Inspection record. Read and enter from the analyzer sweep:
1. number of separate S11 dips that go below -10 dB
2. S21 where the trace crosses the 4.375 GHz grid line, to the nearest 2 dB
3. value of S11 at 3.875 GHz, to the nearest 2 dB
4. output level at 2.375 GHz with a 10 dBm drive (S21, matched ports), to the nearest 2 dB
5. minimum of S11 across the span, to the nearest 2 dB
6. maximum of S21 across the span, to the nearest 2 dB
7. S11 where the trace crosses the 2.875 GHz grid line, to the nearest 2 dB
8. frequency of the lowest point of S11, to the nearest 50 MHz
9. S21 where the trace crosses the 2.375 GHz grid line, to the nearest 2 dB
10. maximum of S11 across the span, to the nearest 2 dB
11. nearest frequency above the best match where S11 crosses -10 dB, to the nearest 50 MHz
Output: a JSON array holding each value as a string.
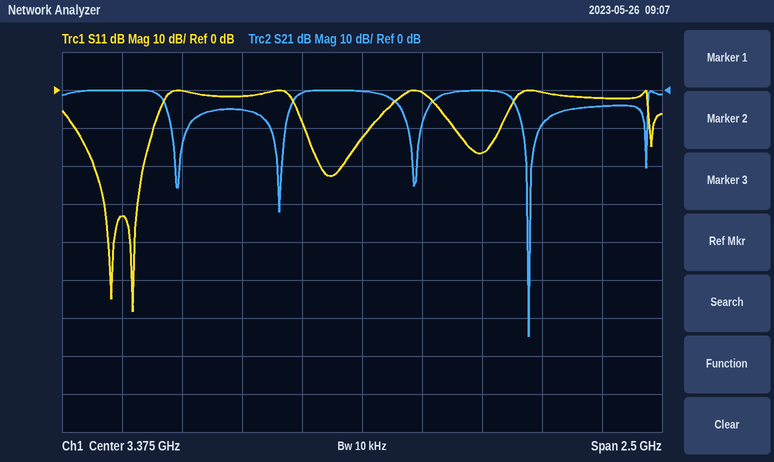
["5", "-4 dB", "-16 dB", "10 dBm", "-58 dB", "0 dB", "-2 dB", "2.40 GHz", "0 dB", "0 dB", "2.50 GHz"]
